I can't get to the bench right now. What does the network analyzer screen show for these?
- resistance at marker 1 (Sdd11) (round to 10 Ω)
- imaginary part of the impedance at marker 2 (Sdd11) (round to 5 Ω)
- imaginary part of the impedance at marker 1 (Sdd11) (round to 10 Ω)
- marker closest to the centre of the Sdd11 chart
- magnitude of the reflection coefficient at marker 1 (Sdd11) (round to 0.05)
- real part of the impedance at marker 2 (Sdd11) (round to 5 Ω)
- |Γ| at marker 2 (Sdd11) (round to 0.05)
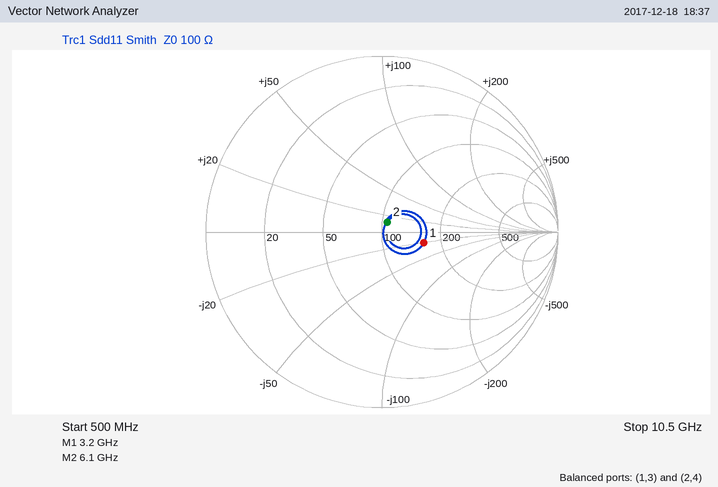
160 Ω
+10 Ω
-20 Ω
marker 2
0.25
105 Ω
0.05
